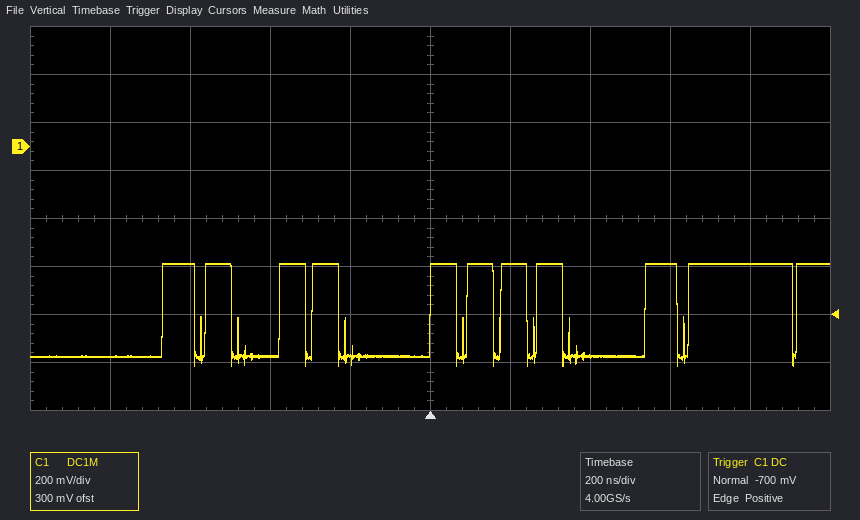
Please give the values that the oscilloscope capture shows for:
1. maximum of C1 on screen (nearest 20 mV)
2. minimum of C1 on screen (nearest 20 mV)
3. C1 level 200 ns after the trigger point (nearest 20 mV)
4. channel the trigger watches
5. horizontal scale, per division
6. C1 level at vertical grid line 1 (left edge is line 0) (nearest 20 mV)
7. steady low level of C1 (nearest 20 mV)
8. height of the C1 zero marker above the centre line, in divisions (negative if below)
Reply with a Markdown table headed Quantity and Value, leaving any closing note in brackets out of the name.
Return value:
| Quantity | Value |
|---|---|
| maximum of C1 on screen | -480 mV |
| minimum of C1 on screen | -920 mV |
| C1 level 200 ns after the trigger point | -480 mV |
| channel the trigger watches | C1 |
| horizontal scale, per division | 200 ns |
| C1 level at vertical grid line 1 (left edge is line 0) | -880 mV |
| steady low level of C1 | -880 mV |
| height of the C1 zero marker above the centre line, in divisions | +1.5 div |
